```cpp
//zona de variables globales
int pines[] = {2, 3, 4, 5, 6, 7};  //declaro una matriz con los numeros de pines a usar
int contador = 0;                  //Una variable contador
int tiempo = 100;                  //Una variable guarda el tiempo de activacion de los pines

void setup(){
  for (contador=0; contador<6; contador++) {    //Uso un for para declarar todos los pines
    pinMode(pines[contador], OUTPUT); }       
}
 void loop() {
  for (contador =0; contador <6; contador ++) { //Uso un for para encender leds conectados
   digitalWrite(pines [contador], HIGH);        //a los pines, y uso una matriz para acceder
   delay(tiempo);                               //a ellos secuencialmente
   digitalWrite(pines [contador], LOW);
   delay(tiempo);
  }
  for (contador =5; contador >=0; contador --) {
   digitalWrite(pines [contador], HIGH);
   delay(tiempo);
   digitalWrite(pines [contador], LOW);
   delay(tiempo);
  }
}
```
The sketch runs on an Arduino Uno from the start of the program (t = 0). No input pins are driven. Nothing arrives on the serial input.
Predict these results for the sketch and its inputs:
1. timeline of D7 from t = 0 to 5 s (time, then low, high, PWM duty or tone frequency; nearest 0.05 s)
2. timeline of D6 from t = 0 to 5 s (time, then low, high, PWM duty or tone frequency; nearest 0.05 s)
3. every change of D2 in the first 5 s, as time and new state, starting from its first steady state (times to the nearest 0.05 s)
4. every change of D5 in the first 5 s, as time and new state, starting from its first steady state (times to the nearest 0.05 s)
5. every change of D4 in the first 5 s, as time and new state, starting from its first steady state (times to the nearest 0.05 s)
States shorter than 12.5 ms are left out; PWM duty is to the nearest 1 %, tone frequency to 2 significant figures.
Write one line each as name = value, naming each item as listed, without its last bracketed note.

timeline of D7 from t = 0 to 5 s = 0 s low; 1 s high; 1.1 s low; 1.2 s high; 1.3 s low; 3.4 s high; 3.5 s low; 3.6 s high; 3.7 s low
timeline of D6 from t = 0 to 5 s = 0 s low; 0.8 s high; 0.9 s low; 1.4 s high; 1.5 s low; 3.2 s high; 3.3 s low; 3.8 s high; 3.9 s low
every change of D2 in the first 5 s, as time and new state, starting from its first steady state = 0 s high; 0.1 s low; 2.2 s high; 2.3 s low; 2.4 s high; 2.5 s low; 4.6 s high; 4.7 s low; 4.8 s high; 4.9 s low
every change of D5 in the first 5 s, as time and new state, starting from its first steady state = 0 s low; 0.6 s high; 0.7 s low; 1.6 s high; 1.7 s low; 3 s high; 3.1 s low; 4 s high; 4.1 s low
every change of D4 in the first 5 s, as time and new state, starting from its first steady state = 0 s low; 0.4 s high; 0.5 s low; 1.8 s high; 1.9 s low; 2.8 s high; 2.9 s low; 4.2 s high; 4.3 s low
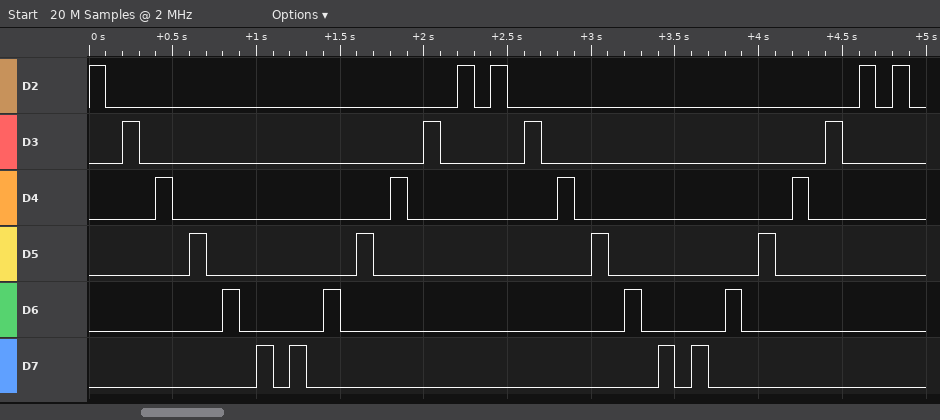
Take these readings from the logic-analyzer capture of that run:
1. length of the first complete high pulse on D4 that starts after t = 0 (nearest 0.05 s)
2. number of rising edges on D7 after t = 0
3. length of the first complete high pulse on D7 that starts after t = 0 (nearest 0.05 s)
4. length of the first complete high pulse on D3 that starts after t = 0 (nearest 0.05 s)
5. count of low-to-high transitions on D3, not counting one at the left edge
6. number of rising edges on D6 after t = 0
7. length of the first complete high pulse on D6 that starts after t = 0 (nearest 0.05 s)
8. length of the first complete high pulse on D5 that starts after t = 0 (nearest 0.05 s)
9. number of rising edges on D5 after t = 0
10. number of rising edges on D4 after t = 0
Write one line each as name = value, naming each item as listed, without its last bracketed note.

length of the first complete high pulse on D4 that starts after t = 0 = 0.10 s
number of rising edges on D7 after t = 0 = 4
length of the first complete high pulse on D7 that starts after t = 0 = 0.10 s
length of the first complete high pulse on D3 that starts after t = 0 = 0.10 s
count of low-to-high transitions on D3, not counting one at the left edge = 4
number of rising edges on D6 after t = 0 = 4
length of the first complete high pulse on D6 that starts after t = 0 = 0.10 s
length of the first complete high pulse on D5 that starts after t = 0 = 0.10 s
number of rising edges on D5 after t = 0 = 4
number of rising edges on D4 after t = 0 = 4
